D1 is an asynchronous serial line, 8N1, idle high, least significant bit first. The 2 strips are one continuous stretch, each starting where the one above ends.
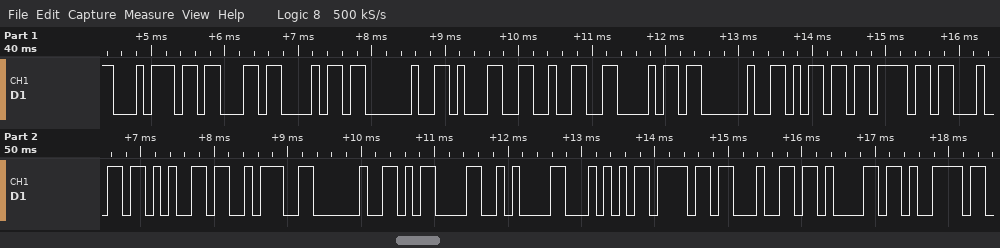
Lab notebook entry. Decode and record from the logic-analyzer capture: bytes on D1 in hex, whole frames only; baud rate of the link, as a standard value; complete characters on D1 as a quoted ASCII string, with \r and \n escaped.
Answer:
74 63 68 20 31 32 68 20 6D 6F 64 65 3A 20 0D 0A 54 6F 64 61 79
9600 baud
"tch 12h mode: \r\nToday"
